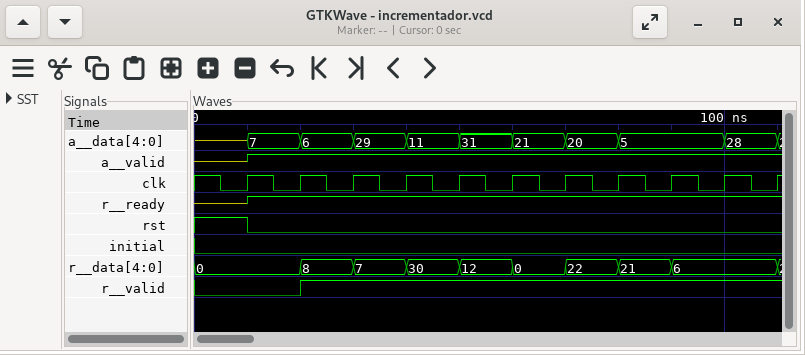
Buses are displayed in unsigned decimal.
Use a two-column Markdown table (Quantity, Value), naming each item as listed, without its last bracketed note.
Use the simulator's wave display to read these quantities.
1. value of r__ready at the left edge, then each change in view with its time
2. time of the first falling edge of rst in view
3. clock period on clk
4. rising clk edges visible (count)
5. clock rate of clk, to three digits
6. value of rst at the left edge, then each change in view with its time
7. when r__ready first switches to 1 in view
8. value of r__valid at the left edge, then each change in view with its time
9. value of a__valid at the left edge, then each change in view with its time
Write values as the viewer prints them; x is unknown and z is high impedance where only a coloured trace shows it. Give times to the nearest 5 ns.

| Quantity | Value |
|---|---|
| value of r__ready at the left edge, then each change in view with its time | z, 1 at 10 ns |
| time of the first falling edge of rst in view | 10 ns |
| clock period on clk | 10 ns |
| rising clk edges visible | 11 |
| clock rate of clk, to three digits | 100 MHz |
| value of rst at the left edge, then each change in view with its time | 1, 0 at 10 ns |
| when r__ready first switches to 1 in view | 10 ns |
| value of r__valid at the left edge, then each change in view with its time | 0, 1 at 20 ns |
| value of a__valid at the left edge, then each change in view with its time | z, 1 at 10 ns |
